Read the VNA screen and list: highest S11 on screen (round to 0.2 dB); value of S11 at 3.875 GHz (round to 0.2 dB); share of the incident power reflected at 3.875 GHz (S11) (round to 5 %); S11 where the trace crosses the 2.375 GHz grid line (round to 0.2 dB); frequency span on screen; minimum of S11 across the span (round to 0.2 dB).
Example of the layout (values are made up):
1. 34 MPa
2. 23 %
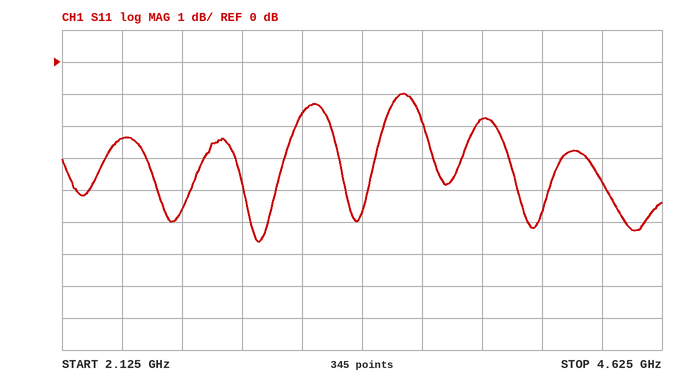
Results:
1. -1.0 dB
2. -1.8 dB
3. 65 %
4. -2.4 dB
5. 2.5 GHz
6. -5.6 dB
